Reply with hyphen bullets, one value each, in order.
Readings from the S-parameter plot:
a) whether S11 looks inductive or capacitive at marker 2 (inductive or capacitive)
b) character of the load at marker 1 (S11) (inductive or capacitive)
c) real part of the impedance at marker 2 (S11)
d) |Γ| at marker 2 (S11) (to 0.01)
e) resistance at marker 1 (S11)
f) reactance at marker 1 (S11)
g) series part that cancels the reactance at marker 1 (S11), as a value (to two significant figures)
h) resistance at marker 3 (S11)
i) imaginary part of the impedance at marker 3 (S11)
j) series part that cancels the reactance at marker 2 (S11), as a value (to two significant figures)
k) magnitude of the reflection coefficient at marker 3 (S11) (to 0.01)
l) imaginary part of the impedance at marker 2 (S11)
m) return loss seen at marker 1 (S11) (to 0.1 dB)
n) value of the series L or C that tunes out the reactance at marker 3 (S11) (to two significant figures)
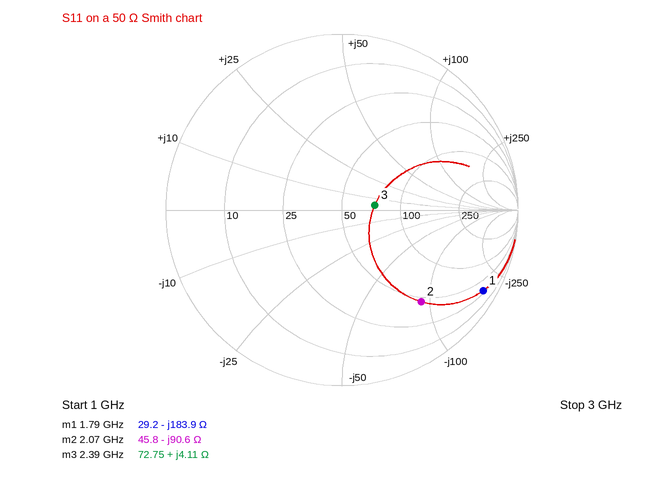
- capacitive
- capacitive
- 45.8 Ω
- 0.69
- 29.2 Ω
- -183.9 Ω
- 16 nH
- 72.75 Ω
- +4.11 Ω
- 7.0 nH
- 0.19
- -90.6 Ω
- 0.7 dB
- 16 pF
